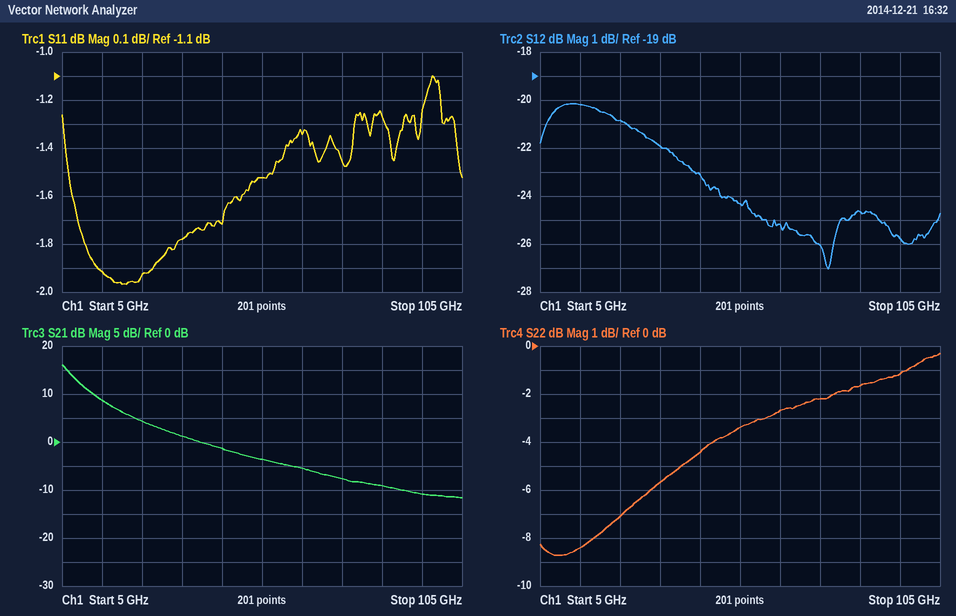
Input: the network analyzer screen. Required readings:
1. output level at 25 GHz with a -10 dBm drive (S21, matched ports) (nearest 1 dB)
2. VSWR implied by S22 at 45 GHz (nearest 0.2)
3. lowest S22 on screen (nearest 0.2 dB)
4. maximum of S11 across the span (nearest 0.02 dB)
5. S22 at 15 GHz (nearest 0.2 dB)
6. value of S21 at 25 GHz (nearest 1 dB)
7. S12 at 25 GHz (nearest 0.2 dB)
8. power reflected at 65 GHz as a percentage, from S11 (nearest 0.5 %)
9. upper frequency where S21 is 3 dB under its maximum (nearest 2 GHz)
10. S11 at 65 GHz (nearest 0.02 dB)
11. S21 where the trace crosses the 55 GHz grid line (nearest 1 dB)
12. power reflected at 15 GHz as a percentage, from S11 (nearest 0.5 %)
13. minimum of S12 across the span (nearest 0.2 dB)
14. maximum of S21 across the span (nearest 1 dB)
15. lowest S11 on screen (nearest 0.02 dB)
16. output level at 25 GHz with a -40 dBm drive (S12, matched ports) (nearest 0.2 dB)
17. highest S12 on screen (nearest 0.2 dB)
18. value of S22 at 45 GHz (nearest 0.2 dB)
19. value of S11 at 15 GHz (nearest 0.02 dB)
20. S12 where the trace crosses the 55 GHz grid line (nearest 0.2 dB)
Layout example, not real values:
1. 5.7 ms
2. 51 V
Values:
1. -6 dBm
2. 4.0
3. -8.8 dB
4. -1.10 dB
5. -8.4 dB
6. 4 dB
7. -20.8 dB
8. 73.5 %
9. 8 GHz
10. -1.34 dB
11. -4 dB
12. 64.5 %
13. -27.0 dB
14. 16 dB
15. -1.96 dB
16. -60.8 dBm
17. -20.2 dB
18. -4.4 dB
19. -1.92 dB
20. -24.4 dB
